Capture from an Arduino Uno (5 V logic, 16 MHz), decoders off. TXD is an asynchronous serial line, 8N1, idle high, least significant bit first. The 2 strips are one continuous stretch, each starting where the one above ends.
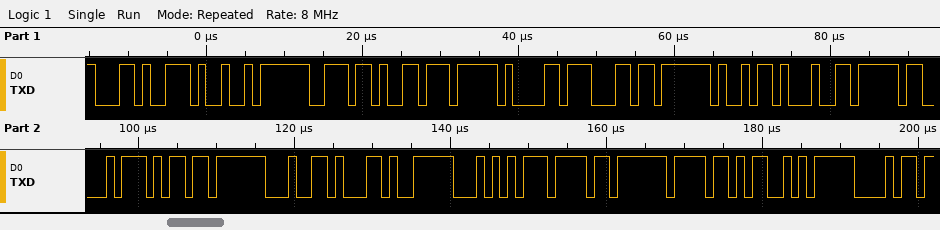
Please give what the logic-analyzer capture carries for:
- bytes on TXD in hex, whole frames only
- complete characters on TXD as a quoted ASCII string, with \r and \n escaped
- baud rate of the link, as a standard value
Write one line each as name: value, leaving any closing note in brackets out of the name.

bytes on TXD in hex, whole frames only: 0x2C 0x49 0x6E 0x76 0x61 0x6C 0x69 0x64 0x43 0x6D 0x64 0x2C 0x54 0x6F 0x6F 0x53 0x68
complete characters on TXD as a quoted ASCII string, with \r and \n escaped: ",InvalidCmd,TooSh"
baud rate of the link, as a standard value: 1000000 baud
